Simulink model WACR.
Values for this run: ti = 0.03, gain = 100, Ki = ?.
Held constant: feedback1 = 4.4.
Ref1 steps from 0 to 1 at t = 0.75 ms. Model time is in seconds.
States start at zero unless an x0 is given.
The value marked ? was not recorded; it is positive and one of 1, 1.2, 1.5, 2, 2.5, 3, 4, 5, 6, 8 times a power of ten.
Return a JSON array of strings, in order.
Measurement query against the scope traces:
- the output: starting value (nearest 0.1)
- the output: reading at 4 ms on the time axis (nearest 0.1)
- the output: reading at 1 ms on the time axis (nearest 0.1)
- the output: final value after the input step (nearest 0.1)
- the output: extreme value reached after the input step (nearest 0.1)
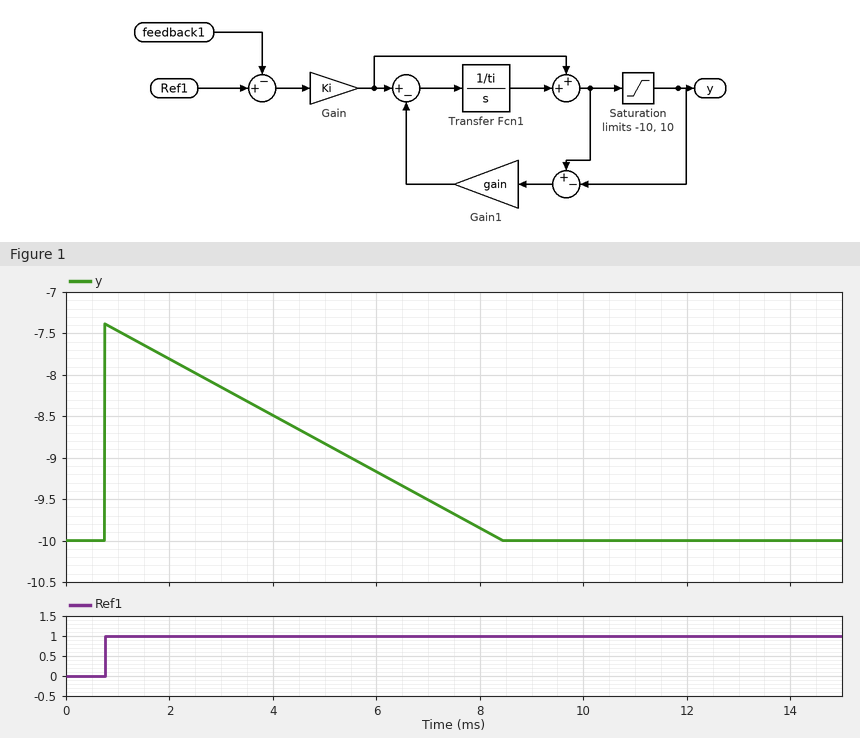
["-10.0", "-8.5", "-7.5", "-10.0", "-7.4"]
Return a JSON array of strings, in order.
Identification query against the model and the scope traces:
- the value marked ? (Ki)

["3"]
